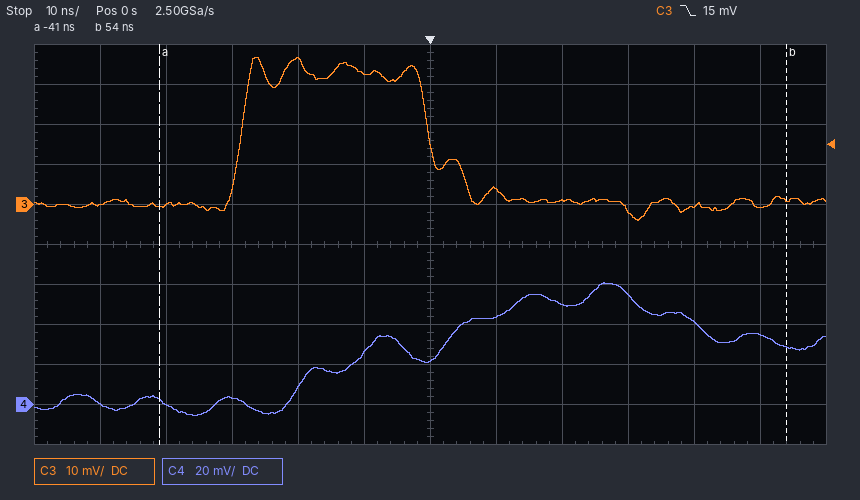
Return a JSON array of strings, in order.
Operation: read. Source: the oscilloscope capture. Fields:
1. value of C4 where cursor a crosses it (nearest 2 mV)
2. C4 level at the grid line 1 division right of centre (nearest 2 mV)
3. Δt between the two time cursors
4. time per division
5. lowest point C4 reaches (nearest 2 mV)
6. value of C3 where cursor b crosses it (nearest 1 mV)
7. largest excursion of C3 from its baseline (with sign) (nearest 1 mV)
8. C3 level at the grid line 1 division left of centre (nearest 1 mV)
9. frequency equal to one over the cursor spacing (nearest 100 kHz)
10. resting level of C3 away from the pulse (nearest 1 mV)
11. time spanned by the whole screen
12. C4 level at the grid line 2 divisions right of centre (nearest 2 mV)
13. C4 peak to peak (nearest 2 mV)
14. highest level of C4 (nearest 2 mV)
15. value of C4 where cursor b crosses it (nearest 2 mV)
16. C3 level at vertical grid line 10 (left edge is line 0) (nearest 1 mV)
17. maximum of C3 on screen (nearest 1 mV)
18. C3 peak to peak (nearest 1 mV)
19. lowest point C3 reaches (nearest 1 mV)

["2 mV", "44 mV", "95 ns", "10 ns", "-6 mV", "1 mV", "+36 mV", "33 mV", "10.5 MHz", "1 mV", "120 ns", "50 mV", "66 mV", "60 mV", "28 mV", "0 mV", "37 mV", "41 mV", "-4 mV"]
